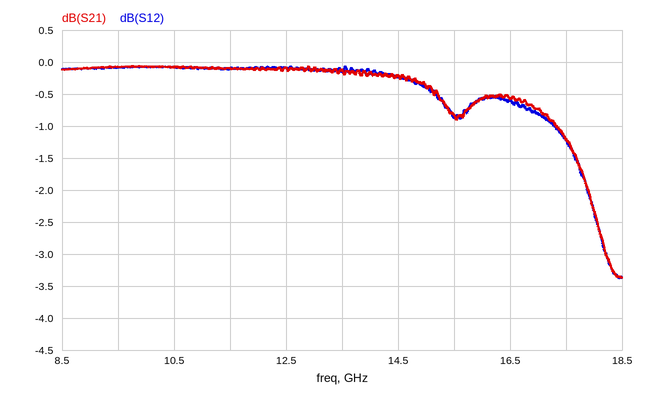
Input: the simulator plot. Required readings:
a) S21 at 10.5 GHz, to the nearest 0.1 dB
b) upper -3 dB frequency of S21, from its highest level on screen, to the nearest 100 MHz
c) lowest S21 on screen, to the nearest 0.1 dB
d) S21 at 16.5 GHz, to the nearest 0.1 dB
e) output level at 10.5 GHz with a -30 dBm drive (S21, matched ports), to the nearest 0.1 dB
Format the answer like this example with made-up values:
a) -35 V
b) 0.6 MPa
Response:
a) -0.1 dB
b) 18.2 GHz
c) -3.4 dB
d) -0.6 dB
e) -30.1 dBm
